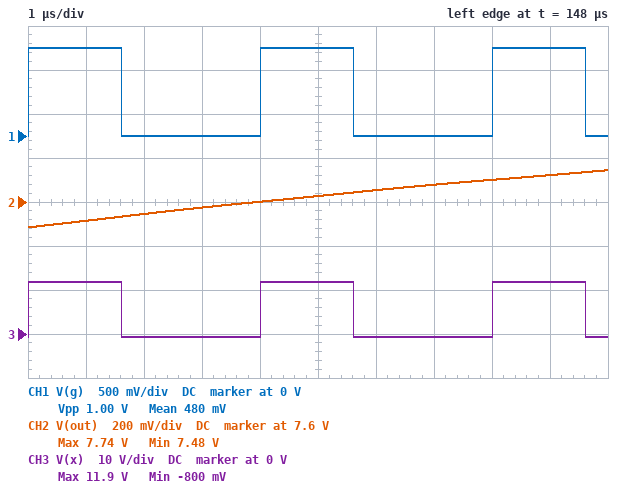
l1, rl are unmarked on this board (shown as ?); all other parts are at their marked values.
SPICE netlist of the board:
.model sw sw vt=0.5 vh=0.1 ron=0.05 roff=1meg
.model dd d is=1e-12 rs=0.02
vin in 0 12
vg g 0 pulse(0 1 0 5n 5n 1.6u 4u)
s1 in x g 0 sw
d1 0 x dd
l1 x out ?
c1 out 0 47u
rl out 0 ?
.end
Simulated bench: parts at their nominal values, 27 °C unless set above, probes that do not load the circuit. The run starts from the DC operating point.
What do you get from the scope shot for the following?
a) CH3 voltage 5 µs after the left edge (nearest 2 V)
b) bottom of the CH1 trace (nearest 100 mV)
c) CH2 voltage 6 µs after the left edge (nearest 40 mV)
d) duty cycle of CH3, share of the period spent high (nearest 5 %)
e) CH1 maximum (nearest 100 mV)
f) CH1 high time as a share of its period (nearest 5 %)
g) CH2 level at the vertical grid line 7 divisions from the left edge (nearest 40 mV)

12 V
0 V
7.64 V
40 %
1.0 V
40 %
7.68 V
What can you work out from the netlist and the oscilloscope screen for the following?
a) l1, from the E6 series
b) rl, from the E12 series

68 µH
12 Ω
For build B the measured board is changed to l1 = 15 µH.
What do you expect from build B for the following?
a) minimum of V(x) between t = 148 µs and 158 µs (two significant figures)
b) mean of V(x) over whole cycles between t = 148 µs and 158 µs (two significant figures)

-710 mV
7.3 V
